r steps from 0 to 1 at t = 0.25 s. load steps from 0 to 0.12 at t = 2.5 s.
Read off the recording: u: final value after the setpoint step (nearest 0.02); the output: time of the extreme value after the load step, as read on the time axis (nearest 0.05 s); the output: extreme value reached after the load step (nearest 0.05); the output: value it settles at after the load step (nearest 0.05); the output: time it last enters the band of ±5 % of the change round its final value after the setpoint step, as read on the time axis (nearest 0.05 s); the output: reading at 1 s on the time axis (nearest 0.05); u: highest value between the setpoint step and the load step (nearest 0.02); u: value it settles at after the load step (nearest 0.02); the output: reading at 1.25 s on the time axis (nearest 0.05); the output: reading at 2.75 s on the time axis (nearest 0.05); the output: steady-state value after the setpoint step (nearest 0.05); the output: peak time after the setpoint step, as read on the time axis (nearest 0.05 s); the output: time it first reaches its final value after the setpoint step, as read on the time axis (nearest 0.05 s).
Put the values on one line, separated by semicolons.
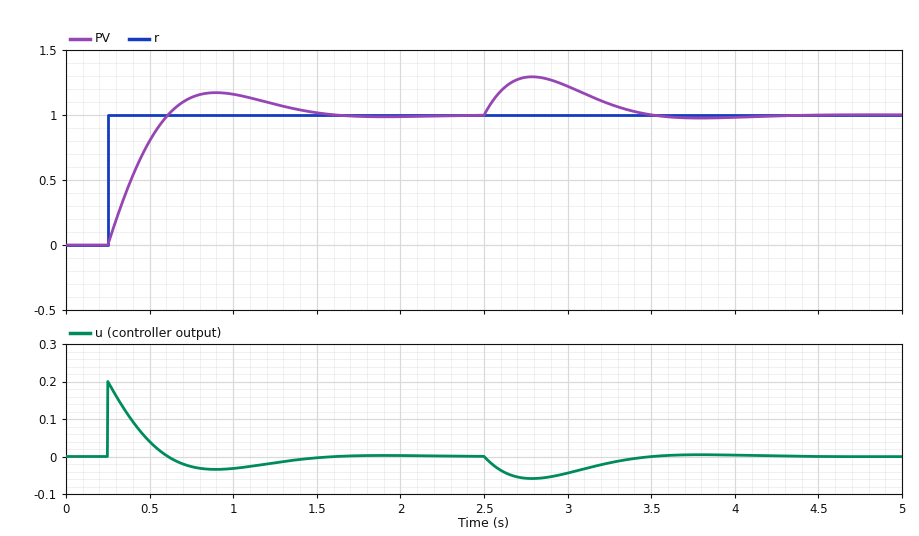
0.00; 2.80 s; 1.30; 1.00; 1.35 s; 1.15; 0.20; 0.00; 1.10; 1.30; 1.00; 0.90 s; 0.60 s
